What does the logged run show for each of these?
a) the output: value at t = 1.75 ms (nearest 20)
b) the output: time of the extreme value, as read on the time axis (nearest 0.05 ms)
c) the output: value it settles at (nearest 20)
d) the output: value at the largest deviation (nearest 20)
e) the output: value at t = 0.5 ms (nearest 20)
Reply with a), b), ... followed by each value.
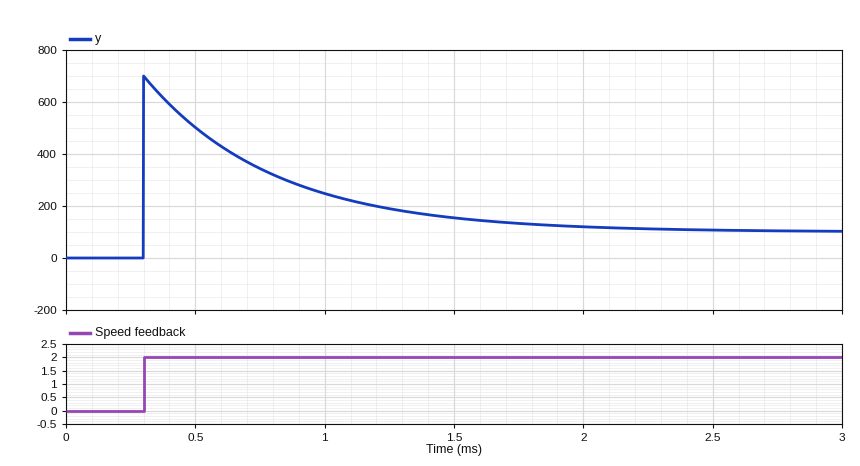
a) 140
b) 0.30 ms
c) 100
d) 700
e) 500
